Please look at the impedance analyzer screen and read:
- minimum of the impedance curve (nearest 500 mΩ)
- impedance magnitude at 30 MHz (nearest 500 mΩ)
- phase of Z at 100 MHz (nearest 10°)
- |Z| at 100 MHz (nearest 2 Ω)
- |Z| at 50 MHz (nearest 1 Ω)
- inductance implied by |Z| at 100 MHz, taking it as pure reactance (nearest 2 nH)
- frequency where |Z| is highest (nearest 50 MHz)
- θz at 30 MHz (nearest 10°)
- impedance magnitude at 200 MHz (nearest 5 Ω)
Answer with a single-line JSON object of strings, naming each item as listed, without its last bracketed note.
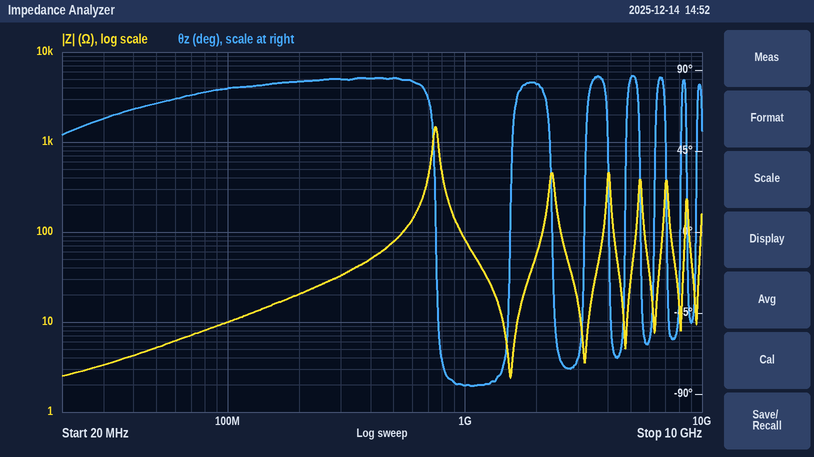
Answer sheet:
{"minimum of the impedance curve": "2.5 Ω", "impedance magnitude at 30 MHz": "3.5 Ω", "phase of Z at 100 MHz": "80°", "|Z| at 100 MHz": "10 Ω", "|Z| at 50 MHz": "5 Ω", "inductance implied by |Z| at 100 MHz, taking it as pure reactance": "16 nH", "frequency where |Z| is highest": "750 MHz", "θz at 30 MHz": "60°", "impedance magnitude at 200 MHz": "20 Ω"}
